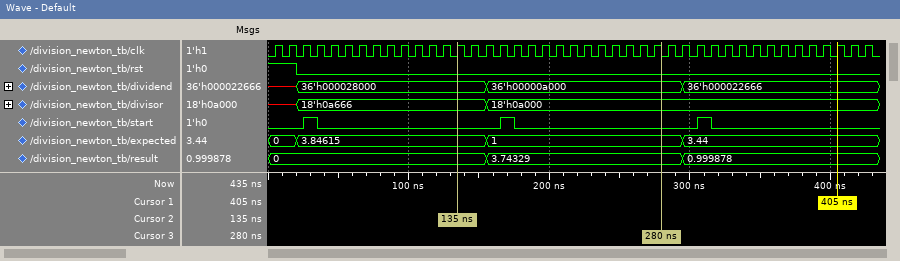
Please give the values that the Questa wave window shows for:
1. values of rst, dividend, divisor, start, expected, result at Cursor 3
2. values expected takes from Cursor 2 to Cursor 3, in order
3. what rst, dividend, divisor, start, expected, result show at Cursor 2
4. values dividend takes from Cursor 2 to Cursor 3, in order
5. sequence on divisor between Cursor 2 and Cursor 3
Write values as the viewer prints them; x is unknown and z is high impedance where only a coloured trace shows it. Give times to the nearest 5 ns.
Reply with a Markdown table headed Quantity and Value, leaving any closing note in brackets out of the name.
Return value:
| Quantity | Value |
|---|---|
| values of rst, dividend, divisor, start, expected, result at Cursor 3 | rst=0, dividend=36'h00000a000, divisor=18'h0a000, start=0, expected=1, result=3.74329 |
| values expected takes from Cursor 2 to Cursor 3, in order | 3.84615, 1 |
| what rst, dividend, divisor, start, expected, result show at Cursor 2 | rst=0, dividend=36'h000028000, divisor=18'h0a666, start=0, expected=3.84615, result=0 |
| values dividend takes from Cursor 2 to Cursor 3, in order | 36'h000028000, 36'h00000a000 |
| sequence on divisor between Cursor 2 and Cursor 3 | 18'h0a666, 18'h0a000 |
